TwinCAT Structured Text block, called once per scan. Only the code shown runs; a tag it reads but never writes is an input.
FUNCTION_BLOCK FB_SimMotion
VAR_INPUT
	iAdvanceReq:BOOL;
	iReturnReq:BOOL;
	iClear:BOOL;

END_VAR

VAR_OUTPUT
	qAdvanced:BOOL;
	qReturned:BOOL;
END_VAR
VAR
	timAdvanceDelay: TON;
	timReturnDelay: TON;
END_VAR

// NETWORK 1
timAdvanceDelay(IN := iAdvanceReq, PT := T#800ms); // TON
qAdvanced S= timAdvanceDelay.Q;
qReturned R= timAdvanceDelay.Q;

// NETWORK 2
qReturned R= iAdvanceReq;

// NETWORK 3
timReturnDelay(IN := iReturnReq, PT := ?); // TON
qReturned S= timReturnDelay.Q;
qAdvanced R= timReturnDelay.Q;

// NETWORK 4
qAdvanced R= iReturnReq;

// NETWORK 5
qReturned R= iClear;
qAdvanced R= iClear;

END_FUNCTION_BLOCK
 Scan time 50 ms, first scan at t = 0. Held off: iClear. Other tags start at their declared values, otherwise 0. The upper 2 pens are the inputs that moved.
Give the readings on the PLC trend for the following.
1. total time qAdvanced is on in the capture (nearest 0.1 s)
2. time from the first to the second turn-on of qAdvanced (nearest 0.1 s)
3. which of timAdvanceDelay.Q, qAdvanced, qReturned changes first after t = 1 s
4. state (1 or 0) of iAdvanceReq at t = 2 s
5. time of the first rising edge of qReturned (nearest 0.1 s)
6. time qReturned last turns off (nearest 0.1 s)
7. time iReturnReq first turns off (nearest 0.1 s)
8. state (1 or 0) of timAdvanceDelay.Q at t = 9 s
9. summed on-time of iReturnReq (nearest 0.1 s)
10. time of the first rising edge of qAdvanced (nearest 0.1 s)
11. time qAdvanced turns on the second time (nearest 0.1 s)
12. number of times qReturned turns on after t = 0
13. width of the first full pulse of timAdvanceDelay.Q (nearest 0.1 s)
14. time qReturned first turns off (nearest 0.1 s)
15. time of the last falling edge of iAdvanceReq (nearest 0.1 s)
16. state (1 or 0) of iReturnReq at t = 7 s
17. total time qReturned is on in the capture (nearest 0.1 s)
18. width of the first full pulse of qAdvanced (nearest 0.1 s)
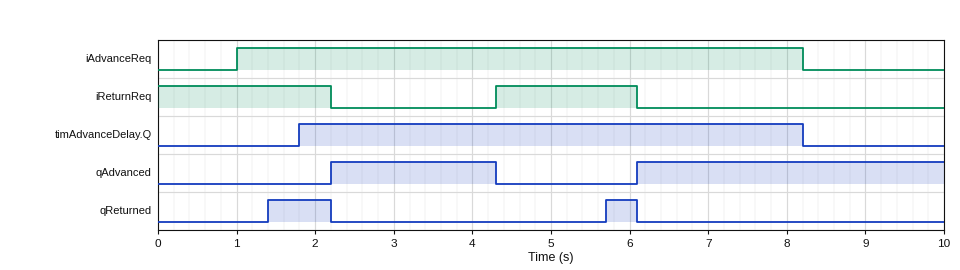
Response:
6.0 s
3.9 s
qReturned
1
1.4 s
6.1 s
2.2 s
0
4.0 s
2.2 s
6.1 s
2
6.4 s
2.2 s
8.2 s
0
1.2 s
2.1 s
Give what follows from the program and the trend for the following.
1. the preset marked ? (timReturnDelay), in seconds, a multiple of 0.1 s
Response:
1.4 s
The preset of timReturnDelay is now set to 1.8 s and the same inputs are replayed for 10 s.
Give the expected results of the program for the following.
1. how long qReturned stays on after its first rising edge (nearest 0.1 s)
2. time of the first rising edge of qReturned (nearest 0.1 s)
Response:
0.4 s
1.8 s
